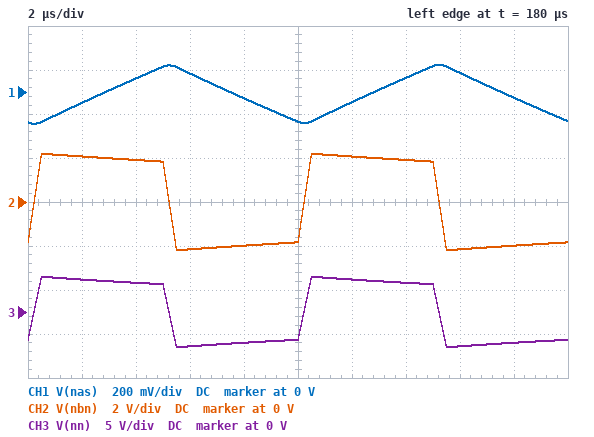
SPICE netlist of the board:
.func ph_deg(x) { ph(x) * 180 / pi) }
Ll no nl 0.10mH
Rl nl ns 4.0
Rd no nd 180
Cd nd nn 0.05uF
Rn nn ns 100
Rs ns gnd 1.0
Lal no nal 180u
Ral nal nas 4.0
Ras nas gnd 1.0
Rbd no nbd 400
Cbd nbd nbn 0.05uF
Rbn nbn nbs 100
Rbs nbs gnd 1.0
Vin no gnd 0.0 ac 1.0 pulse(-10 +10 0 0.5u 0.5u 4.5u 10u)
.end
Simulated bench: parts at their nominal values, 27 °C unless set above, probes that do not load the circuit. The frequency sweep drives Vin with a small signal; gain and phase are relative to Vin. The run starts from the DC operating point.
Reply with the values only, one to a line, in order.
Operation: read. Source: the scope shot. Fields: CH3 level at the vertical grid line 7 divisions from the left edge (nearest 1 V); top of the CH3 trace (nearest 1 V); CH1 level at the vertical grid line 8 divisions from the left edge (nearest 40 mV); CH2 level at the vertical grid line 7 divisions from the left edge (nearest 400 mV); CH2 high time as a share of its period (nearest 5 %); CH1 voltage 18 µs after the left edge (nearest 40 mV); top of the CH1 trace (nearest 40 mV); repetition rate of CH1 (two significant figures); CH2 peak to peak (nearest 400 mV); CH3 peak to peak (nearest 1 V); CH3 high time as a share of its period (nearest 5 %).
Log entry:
3 V
4 V
80 mV
2.0 V
50 %
-40 mV
120 mV
100 kHz
4.4 V
8 V
50 %
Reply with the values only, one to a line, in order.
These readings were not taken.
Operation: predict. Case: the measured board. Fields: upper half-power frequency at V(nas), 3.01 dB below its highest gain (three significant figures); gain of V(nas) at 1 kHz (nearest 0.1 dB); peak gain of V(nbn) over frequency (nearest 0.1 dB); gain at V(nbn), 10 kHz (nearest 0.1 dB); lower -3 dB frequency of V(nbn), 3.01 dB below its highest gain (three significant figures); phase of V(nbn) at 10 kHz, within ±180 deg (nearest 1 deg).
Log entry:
4.42 kHz
-14.2 dB
-13.9 dB
-15.4 dB
6.35 kHz
32 deg
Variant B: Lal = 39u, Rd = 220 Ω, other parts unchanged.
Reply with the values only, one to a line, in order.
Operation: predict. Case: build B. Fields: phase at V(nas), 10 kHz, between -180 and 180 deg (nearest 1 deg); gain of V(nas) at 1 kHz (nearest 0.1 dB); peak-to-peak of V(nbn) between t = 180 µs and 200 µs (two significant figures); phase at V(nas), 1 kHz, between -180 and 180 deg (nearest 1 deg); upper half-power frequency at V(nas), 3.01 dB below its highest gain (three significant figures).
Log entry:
-26 deg
-14.0 dB
4.4 V
-3 deg
20.4 kHz
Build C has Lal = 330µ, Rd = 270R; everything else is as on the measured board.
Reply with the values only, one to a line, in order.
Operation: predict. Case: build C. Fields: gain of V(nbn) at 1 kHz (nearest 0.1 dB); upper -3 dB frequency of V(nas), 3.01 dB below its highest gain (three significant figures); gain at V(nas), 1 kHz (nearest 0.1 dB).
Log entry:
-30.1 dB
2.41 kHz
-14.7 dB
